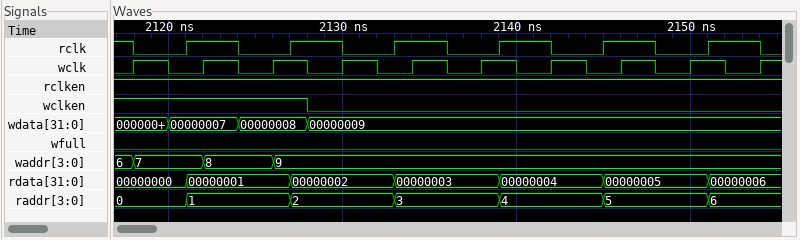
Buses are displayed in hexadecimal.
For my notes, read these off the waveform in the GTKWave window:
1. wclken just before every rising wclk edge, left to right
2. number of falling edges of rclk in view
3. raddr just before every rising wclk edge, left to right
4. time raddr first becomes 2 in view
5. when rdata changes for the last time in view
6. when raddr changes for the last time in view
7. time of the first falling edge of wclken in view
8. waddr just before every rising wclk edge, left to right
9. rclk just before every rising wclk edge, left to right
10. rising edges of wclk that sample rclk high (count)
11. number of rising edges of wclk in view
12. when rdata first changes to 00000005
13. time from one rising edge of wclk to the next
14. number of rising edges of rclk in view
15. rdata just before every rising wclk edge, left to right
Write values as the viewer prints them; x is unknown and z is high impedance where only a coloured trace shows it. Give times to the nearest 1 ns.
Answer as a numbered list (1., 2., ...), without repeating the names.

1. 1 1 1 0 0 0 0 0 0 0
2. 7
3. 0, 1, 1, 2, 3, 3, 4, 5, 5, 6
4. 2127 ns
5. 2151 ns
6. 2151 ns
7. 2128 ns
8. 6, 7, 8, 9, 9, 9, 9, 9, 9, 9
9. 1 1 0 1 1 0 1 1 0 1
10. 7
11. 10
12. 2145 ns
13. 4 ns
14. 6
15. 00000000, 00000001, 00000001, 00000002, 00000003, 00000003, 00000004, 00000005, 00000005, 00000006
